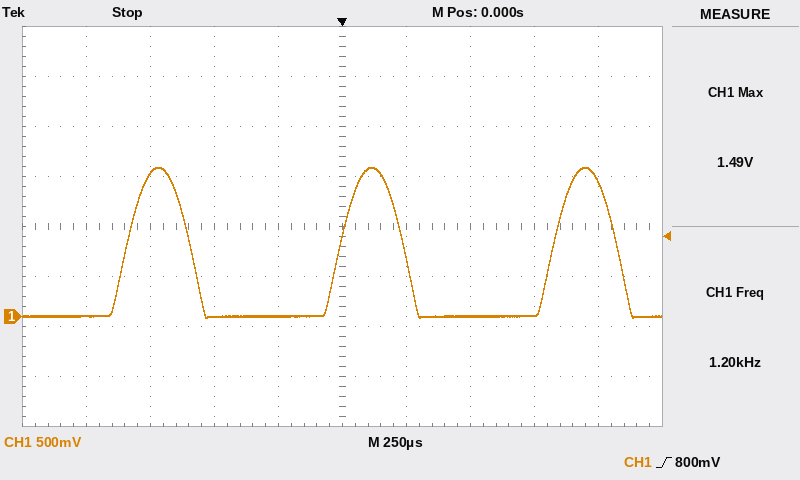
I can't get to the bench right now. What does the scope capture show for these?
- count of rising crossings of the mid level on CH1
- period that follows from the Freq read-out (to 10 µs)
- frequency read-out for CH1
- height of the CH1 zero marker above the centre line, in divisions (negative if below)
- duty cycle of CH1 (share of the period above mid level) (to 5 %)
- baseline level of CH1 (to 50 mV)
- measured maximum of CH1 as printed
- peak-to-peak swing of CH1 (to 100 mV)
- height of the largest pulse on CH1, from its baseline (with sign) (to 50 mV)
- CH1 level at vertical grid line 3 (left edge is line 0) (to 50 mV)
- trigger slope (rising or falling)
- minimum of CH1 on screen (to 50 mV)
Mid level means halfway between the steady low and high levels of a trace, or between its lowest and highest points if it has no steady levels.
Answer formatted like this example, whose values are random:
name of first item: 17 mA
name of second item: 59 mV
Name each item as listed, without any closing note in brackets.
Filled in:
count of rising crossings of the mid level on CH1: 3
period that follows from the Freq read-out: 830 µs
frequency read-out for CH1: 1.20 kHz
height of the CH1 zero marker above the centre line, in divisions: -1.8 div
duty cycle of CH1 (share of the period above mid level): 30 %
baseline level of CH1: 0 mV
measured maximum of CH1 as printed: 1.49 V
peak-to-peak swing of CH1: 1.50 V
height of the largest pulse on CH1, from its baseline (with sign): +1.50 V
CH1 level at vertical grid line 3 (left edge is line 0): 0 mV
trigger slope: rising
minimum of CH1 on screen: 0 mV
